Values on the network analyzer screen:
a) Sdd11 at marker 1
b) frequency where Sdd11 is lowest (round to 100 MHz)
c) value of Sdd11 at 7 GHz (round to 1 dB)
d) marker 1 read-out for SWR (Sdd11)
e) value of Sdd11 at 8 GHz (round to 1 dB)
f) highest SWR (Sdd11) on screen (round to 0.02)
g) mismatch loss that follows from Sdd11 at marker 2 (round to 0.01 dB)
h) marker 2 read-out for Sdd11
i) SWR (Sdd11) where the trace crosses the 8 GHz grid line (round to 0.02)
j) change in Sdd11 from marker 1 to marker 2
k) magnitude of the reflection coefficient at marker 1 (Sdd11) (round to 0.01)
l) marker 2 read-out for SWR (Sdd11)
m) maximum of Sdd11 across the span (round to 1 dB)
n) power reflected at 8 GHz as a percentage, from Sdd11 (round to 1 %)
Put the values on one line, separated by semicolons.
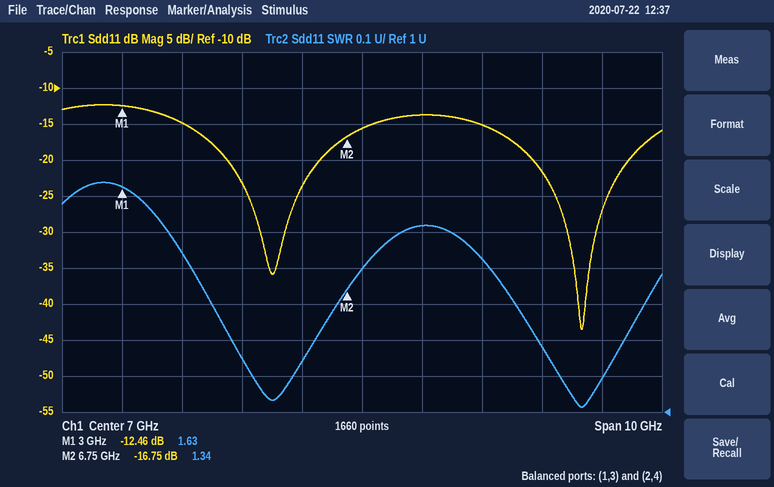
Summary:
-12.46 dB; 10.7 GHz; -16 dB; 1.63; -14 dB; 1.64; 0.09 dB; -16.75 dB; 1.52; -4.29 dB; 0.24; 1.34; -12 dB; 4 %
